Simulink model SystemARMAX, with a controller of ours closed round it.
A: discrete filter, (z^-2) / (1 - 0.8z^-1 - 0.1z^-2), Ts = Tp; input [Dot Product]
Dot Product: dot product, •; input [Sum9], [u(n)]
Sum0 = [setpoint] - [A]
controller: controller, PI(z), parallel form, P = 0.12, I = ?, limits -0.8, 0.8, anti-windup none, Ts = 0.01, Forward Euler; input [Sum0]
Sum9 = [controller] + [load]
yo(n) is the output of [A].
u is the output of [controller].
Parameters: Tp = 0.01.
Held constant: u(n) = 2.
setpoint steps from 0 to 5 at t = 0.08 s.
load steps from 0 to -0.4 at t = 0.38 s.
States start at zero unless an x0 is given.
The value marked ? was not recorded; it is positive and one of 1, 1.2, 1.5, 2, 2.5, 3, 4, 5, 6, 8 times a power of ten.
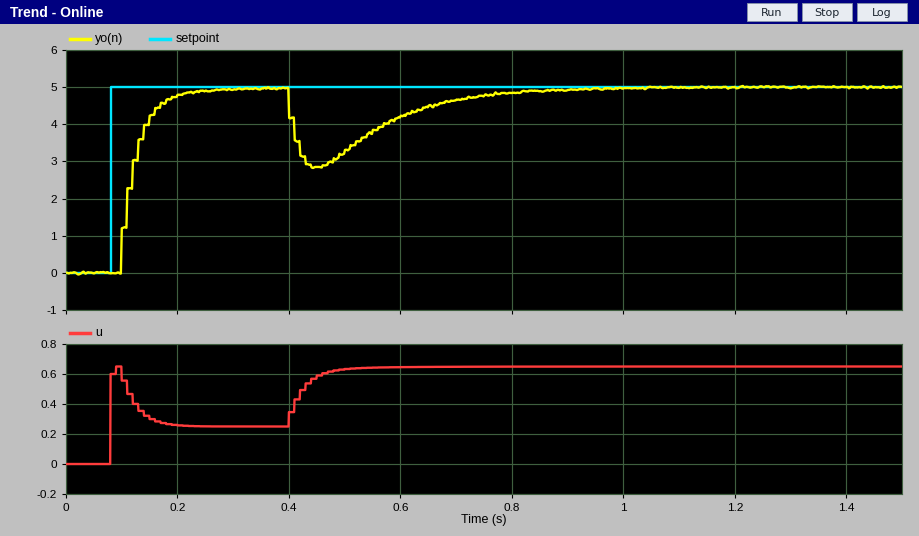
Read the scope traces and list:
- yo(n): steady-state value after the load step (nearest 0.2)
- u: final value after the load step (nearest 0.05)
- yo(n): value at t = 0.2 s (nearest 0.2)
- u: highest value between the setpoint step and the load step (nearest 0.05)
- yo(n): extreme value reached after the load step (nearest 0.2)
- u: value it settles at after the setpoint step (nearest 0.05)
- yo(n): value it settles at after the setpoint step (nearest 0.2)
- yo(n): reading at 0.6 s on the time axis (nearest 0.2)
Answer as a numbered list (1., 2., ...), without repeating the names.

1. 5.0
2. 0.65
3. 4.8
4. 0.65
5. 2.8
6. 0.25
7. 5.0
8. 4.2
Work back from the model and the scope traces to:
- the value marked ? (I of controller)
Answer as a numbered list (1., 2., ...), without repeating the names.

1. 1
